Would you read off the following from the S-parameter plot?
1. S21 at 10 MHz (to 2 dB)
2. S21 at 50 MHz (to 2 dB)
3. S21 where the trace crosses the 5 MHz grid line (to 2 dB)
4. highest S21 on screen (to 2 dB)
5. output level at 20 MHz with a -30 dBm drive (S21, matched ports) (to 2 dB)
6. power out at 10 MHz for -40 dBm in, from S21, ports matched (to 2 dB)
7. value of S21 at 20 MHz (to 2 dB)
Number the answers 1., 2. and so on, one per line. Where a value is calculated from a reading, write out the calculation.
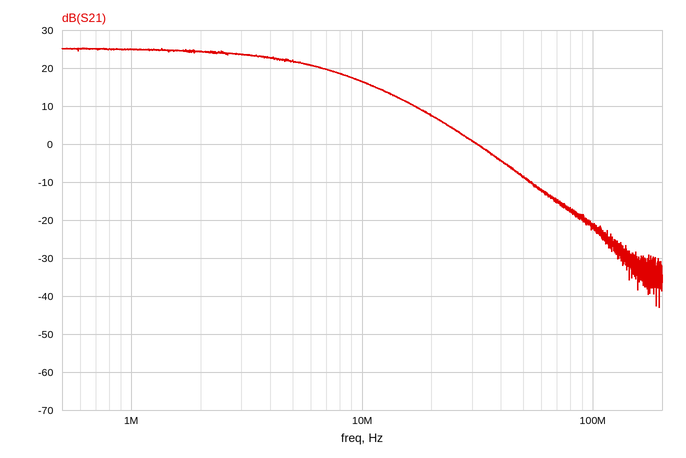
1. 16 dB
2. -8 dB
3. 22 dB
4. 26 dB
5. -30 dBm + (8 dB) = -22 dBm
6. -40 dBm + (16 dB) = -24 dBm
7. 8 dB
